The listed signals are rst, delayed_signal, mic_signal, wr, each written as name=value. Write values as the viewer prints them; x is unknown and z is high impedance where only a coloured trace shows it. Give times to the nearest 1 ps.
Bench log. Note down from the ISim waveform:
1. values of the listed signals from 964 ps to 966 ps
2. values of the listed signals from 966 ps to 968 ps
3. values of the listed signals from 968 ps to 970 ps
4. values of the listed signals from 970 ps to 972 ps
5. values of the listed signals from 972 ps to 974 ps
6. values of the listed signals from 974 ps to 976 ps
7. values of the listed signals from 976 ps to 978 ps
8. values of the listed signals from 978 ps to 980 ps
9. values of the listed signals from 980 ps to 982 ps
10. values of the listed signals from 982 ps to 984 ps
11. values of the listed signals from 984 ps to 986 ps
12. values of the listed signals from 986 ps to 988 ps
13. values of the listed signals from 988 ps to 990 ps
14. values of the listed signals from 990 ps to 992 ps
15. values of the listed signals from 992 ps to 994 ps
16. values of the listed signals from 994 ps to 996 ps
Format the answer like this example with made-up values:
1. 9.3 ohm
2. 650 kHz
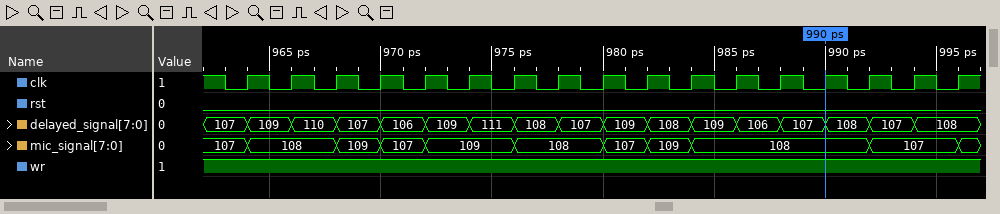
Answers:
1. rst=0, delayed_signal=109, mic_signal=108, wr=1
2. rst=0, delayed_signal=110, mic_signal=108, wr=1
3. rst=0, delayed_signal=107, mic_signal=109, wr=1
4. rst=0, delayed_signal=106, mic_signal=107, wr=1
5. rst=0, delayed_signal=109, mic_signal=109, wr=1
6. rst=0, delayed_signal=111, mic_signal=109, wr=1
7. rst=0, delayed_signal=108, mic_signal=108, wr=1
8. rst=0, delayed_signal=107, mic_signal=108, wr=1
9. rst=0, delayed_signal=109, mic_signal=107, wr=1
10. rst=0, delayed_signal=108, mic_signal=109, wr=1
11. rst=0, delayed_signal=109, mic_signal=108, wr=1
12. rst=0, delayed_signal=106, mic_signal=108, wr=1
13. rst=0, delayed_signal=107, mic_signal=108, wr=1
14. rst=0, delayed_signal=108, mic_signal=108, wr=1
15. rst=0, delayed_signal=107, mic_signal=107, wr=1
16. rst=0, delayed_signal=108, mic_signal=107, wr=1
